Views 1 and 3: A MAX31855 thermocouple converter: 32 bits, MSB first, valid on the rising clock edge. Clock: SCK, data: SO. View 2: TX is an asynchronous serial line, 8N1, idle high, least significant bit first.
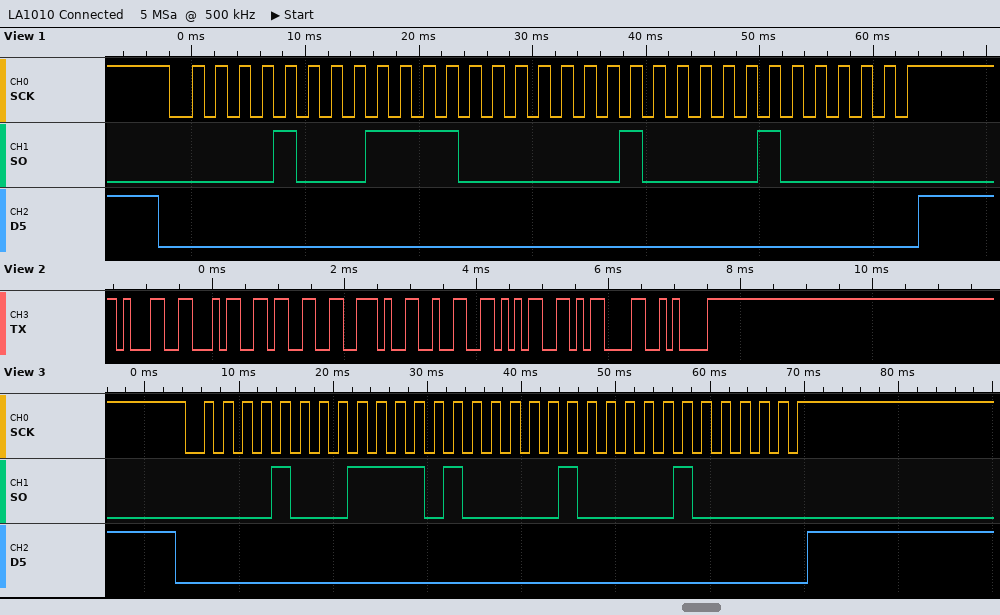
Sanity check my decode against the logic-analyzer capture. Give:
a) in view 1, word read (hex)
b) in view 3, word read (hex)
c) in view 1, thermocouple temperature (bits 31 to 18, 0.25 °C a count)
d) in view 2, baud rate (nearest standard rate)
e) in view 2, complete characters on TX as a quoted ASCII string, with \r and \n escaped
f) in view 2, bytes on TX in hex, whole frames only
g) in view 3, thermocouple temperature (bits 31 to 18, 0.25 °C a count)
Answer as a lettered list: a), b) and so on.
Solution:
a) 0x08F01040
b) 0x08F41040
c) 143.00 °C
d) 9600 baud
e) "143.25\r\n"
f) 31 34 33 2E 32 35 0D 0A
g) 143.25 °C
